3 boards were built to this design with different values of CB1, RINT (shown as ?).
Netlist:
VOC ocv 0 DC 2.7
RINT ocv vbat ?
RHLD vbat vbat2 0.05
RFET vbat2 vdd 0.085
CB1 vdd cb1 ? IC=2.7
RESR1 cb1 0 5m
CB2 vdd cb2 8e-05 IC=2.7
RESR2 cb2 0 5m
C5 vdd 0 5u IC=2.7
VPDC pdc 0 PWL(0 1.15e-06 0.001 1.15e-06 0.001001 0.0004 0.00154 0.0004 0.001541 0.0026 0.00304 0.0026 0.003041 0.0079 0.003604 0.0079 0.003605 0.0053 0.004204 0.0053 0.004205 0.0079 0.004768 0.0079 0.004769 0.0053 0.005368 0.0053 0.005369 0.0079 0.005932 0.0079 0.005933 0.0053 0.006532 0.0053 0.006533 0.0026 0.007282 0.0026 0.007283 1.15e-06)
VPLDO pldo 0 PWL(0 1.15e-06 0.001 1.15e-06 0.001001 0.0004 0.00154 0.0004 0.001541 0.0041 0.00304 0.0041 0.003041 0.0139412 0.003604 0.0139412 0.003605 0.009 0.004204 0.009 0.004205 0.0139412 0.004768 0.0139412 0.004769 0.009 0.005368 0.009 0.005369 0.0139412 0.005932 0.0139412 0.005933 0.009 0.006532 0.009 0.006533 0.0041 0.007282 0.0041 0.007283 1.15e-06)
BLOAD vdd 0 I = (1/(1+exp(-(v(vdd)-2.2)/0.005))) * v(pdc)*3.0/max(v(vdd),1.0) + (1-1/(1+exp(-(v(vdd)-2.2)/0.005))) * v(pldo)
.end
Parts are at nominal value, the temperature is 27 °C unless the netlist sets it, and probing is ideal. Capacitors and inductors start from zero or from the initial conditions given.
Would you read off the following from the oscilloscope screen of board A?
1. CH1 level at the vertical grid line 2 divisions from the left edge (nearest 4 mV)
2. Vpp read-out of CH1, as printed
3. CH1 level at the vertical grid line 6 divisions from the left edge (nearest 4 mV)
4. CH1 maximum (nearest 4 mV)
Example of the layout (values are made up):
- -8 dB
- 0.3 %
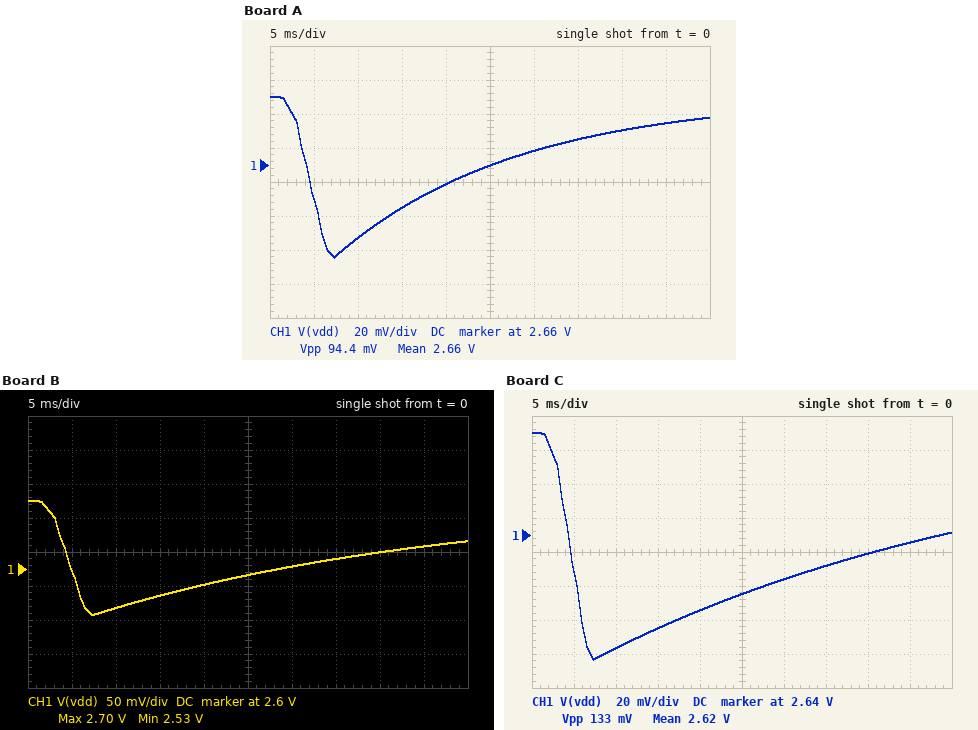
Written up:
- 2.616 V
- 94.4 mV
- 2.668 V
- 2.700 V
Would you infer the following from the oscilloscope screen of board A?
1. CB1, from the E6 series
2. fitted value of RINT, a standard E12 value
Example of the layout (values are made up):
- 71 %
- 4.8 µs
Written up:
- 220 µF
- 68 Ω
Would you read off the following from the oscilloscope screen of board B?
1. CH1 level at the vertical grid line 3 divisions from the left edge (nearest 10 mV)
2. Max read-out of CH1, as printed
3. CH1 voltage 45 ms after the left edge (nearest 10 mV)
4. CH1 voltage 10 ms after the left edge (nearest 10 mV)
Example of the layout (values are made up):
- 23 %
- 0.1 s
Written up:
- 2.56 V
- 2.70 V
- 2.63 V
- 2.54 V
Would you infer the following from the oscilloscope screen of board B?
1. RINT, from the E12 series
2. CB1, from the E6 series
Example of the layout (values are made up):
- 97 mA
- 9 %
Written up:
- 220 Ω
- 100 µF
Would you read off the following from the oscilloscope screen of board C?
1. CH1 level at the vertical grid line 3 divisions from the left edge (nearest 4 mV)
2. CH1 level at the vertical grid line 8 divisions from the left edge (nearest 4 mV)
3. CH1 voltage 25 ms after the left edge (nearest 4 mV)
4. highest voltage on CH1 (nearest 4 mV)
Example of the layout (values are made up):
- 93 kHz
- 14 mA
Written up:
- 2.584 V
- 2.628 V
- 2.604 V
- 2.700 V
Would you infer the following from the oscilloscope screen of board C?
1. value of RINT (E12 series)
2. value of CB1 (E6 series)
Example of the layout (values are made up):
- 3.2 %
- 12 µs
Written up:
- 220 Ω
- 150 µF
